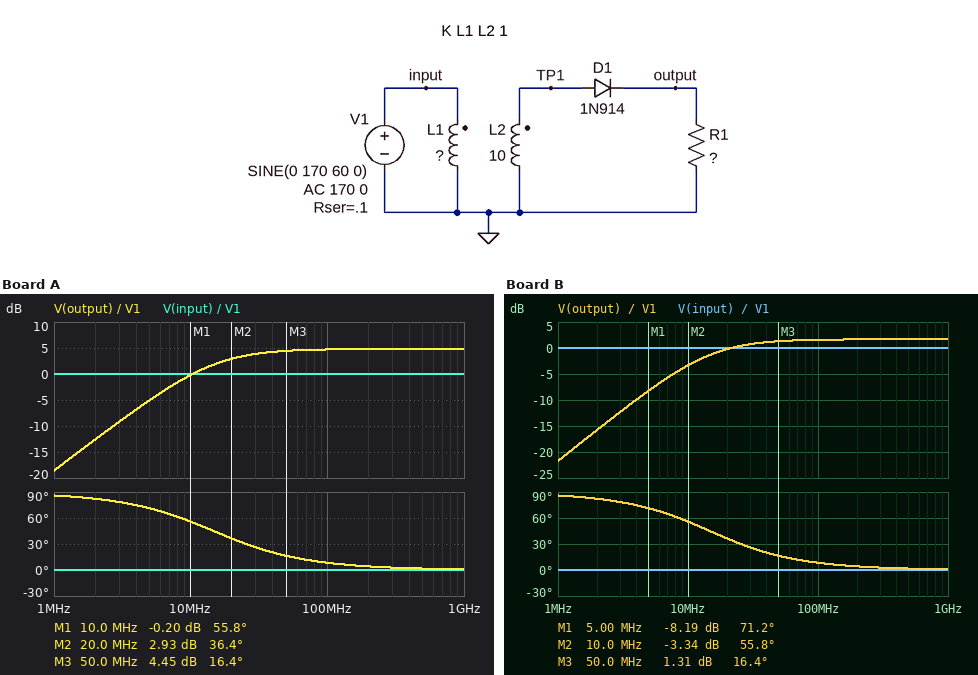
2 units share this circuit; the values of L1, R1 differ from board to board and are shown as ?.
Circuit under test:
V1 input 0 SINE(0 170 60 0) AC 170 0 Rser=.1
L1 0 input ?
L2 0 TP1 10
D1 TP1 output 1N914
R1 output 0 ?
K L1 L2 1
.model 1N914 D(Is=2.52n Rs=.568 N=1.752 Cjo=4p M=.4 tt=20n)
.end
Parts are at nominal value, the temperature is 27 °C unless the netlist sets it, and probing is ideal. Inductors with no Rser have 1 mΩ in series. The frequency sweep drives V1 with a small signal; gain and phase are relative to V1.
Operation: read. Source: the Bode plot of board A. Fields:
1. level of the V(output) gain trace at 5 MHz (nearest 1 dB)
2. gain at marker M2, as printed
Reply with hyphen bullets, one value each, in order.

- -5 dB
- 2.93 dB
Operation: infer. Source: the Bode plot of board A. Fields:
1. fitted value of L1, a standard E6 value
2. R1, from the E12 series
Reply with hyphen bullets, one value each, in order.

- 3.3 H
- 2.7 kΩ
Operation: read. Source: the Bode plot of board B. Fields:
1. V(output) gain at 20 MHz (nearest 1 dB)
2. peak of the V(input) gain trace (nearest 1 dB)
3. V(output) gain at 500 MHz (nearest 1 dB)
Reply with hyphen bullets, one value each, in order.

- 0 dB
- 0 dB
- 2 dB
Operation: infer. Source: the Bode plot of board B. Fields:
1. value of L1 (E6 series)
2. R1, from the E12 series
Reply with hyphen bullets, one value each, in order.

- 6.8 H
- 2.7 kΩ
